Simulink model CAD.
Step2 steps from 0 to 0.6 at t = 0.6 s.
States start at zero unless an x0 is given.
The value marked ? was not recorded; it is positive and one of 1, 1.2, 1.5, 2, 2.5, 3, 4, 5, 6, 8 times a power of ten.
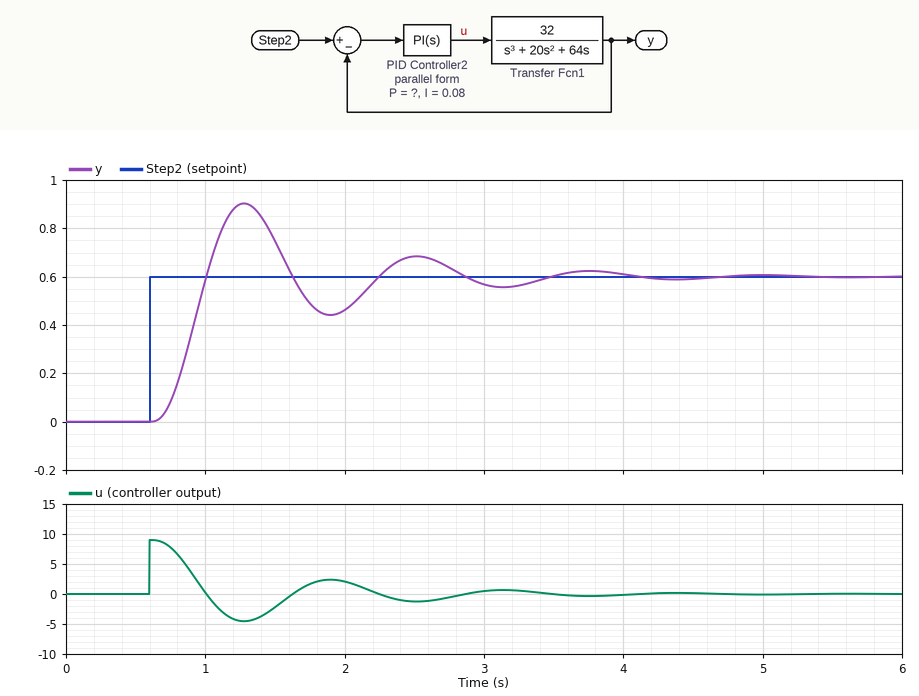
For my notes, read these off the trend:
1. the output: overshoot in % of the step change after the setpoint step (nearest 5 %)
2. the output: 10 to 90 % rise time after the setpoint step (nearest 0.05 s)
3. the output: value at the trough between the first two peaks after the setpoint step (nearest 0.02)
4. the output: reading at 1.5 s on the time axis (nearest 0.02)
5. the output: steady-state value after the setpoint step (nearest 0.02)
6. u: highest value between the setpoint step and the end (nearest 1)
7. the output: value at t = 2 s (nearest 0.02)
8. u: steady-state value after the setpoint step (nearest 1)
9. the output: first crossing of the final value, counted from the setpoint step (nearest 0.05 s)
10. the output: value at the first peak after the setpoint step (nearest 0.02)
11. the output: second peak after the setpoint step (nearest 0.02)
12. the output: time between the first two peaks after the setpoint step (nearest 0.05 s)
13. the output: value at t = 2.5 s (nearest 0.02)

50 %
0.25 s
0.44
0.74
0.60
9
0.46
0
0.40 s
0.90
0.68
1.25 s
0.68
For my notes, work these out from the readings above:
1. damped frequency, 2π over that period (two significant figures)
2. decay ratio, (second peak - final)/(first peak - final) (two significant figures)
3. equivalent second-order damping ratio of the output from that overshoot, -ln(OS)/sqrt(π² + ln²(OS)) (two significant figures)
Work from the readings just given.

5.0 rad/s
0.27
0.22
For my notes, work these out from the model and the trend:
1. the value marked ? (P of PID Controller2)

15
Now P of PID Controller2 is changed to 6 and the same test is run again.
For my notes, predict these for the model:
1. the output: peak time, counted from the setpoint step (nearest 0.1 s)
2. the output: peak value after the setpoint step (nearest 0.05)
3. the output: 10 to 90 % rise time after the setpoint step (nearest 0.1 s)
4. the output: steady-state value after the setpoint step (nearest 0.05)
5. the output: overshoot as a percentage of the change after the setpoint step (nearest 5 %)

1.1 s
0.70
0.5 s
0.60
20 %
